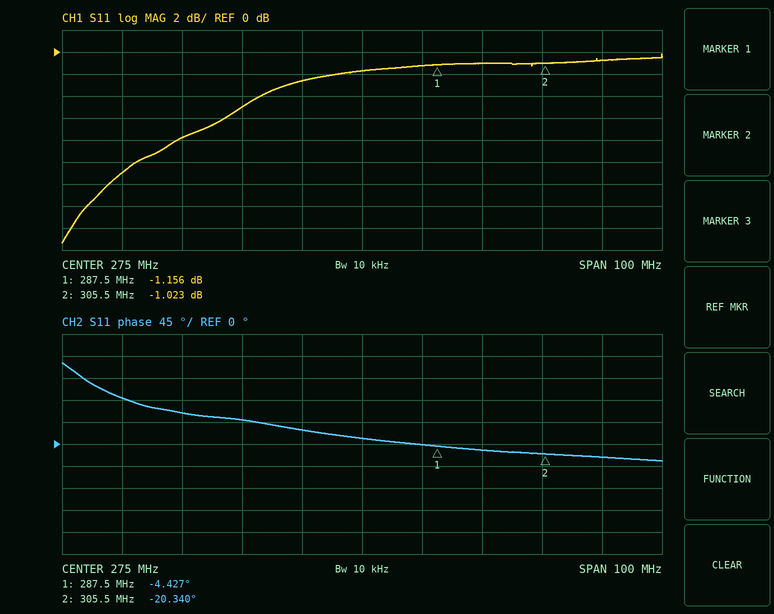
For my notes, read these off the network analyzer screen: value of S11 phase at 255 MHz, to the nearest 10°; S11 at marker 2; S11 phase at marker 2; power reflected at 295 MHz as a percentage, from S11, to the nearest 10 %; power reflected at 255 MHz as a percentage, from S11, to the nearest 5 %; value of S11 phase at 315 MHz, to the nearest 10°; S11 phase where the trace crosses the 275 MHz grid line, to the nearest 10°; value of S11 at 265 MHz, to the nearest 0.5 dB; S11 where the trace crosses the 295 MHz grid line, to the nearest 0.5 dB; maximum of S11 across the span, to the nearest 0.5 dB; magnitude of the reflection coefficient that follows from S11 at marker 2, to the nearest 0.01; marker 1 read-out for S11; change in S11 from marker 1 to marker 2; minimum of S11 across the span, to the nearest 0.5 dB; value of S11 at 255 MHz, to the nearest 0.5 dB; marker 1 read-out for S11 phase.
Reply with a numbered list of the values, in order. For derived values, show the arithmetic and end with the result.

1. 50°
2. -1.023 dB
3. -20.340°
4. 10^(-1/10) ≈ 79.4 %, so 80 % to the nearest 10 %
5. 10^(-5/10) ≈ 31.6 %, so 30 % to the nearest 5 %
6. -30°
7. 10°
8. -2.5 dB
9. -1.0 dB
10. 0.0 dB
11. 10^(-1.023/20) ≈ 0.89
12. -1.156 dB
13. -1.023 − (-1.156) = 0.133 dB
14. -17.5 dB
15. -5.0 dB
16. -4.427°
